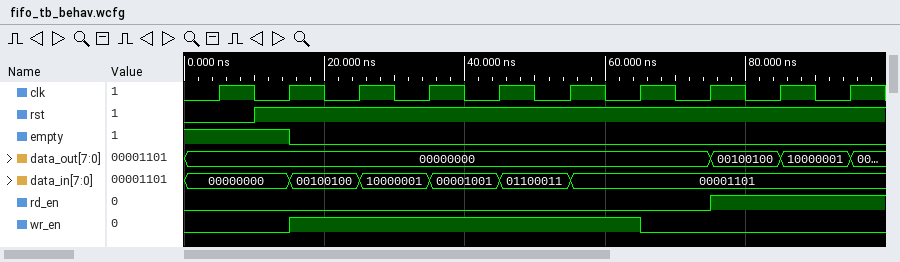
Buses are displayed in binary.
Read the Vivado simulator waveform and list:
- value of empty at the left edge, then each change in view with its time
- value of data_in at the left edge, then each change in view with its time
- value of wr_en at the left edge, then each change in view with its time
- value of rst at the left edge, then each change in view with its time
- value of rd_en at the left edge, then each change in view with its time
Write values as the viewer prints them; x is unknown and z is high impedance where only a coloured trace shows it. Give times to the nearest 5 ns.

1, 0 at 15 ns
00000000, 00100100 at 15 ns, 10000001 at 25 ns, 00001001 at 35 ns, 01100011 at 45 ns, 00001101 at 55 ns
0, 1 at 15 ns, 0 at 65 ns
0, 1 at 10 ns
0, 1 at 75 ns
